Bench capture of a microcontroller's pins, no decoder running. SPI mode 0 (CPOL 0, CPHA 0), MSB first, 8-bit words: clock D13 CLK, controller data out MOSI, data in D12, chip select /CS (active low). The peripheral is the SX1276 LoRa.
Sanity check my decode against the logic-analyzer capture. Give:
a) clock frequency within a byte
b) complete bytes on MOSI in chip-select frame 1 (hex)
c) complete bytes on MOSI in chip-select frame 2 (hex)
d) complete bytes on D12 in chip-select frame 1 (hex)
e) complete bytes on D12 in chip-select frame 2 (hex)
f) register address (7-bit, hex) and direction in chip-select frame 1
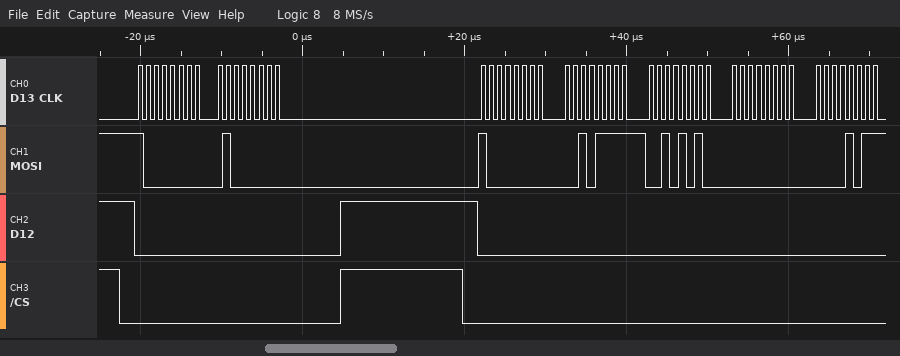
1 MHz
80 40
80 2F 2A 00 0B
00 00
00 00 00 00 00
0x00 write
